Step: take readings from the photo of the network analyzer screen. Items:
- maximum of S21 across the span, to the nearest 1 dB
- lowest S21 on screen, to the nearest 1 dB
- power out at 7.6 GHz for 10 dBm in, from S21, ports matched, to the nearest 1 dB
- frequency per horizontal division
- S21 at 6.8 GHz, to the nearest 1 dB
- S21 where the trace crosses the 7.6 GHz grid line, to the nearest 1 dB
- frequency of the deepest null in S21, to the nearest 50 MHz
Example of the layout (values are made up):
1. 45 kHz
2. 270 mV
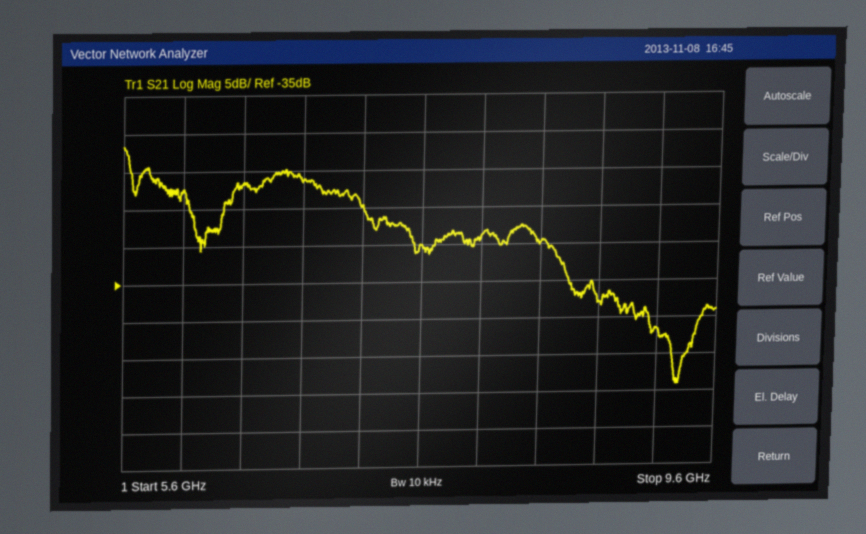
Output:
1. -17 dB
2. -49 dB
3. -20 dBm
4. 400 MHz
5. -21 dB
6. -30 dB
7. 9.35 GHz
